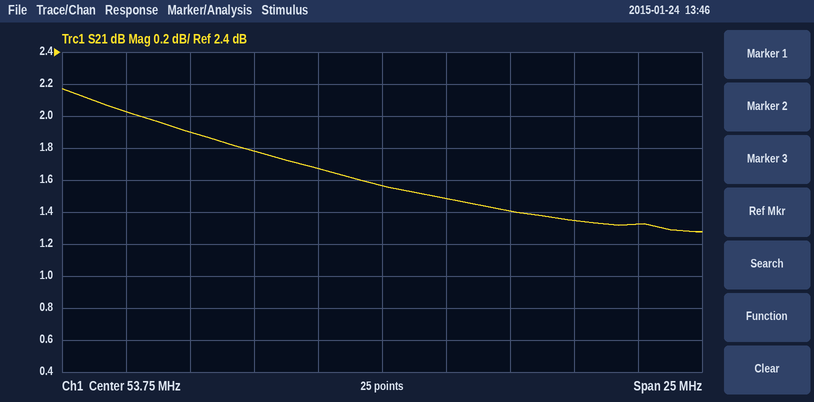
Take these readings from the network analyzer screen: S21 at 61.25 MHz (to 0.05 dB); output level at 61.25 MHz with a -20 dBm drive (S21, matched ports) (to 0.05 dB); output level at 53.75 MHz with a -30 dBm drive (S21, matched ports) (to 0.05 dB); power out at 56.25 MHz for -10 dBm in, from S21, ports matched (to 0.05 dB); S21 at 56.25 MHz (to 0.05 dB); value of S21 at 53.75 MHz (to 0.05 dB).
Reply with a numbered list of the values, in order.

1. 1.35 dB
2. -18.65 dBm
3. -28.45 dBm
4. -8.50 dBm
5. 1.50 dB
6. 1.55 dB
